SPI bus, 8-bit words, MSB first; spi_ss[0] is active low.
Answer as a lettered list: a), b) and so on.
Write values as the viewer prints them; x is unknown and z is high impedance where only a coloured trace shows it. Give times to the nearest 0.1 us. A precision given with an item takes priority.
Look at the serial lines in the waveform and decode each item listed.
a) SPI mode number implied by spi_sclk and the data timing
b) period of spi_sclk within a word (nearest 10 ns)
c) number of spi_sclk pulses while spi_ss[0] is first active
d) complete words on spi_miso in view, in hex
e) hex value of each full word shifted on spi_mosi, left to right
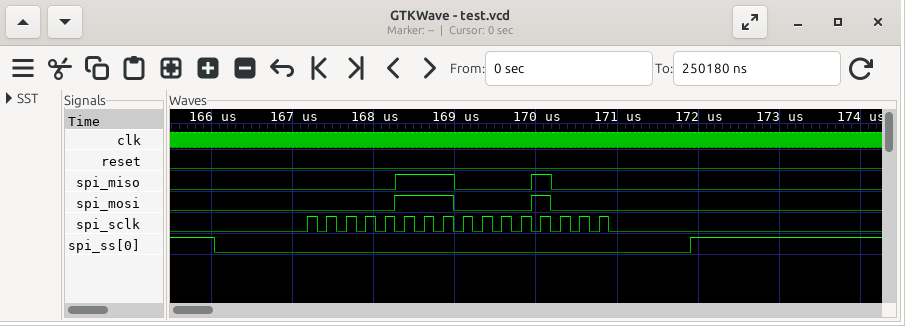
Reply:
a) 0
b) 240 ns
c) 16
d) 07, 08
e) 07, 08
